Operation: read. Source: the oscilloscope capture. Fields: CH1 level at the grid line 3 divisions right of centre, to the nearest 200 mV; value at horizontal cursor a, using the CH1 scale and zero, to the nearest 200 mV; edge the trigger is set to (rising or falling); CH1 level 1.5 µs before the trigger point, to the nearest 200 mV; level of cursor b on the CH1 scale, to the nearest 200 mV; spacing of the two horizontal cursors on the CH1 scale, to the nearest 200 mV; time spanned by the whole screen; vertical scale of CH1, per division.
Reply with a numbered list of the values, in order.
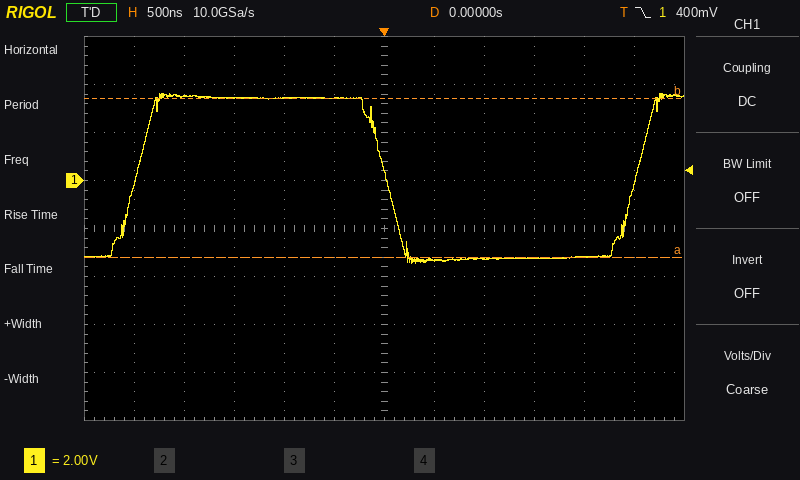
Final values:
1. -3.2 V
2. -3.2 V
3. falling
4. 3.4 V
5. 3.4 V
6. 6.6 V
7. 6 µs
8. 2 V
